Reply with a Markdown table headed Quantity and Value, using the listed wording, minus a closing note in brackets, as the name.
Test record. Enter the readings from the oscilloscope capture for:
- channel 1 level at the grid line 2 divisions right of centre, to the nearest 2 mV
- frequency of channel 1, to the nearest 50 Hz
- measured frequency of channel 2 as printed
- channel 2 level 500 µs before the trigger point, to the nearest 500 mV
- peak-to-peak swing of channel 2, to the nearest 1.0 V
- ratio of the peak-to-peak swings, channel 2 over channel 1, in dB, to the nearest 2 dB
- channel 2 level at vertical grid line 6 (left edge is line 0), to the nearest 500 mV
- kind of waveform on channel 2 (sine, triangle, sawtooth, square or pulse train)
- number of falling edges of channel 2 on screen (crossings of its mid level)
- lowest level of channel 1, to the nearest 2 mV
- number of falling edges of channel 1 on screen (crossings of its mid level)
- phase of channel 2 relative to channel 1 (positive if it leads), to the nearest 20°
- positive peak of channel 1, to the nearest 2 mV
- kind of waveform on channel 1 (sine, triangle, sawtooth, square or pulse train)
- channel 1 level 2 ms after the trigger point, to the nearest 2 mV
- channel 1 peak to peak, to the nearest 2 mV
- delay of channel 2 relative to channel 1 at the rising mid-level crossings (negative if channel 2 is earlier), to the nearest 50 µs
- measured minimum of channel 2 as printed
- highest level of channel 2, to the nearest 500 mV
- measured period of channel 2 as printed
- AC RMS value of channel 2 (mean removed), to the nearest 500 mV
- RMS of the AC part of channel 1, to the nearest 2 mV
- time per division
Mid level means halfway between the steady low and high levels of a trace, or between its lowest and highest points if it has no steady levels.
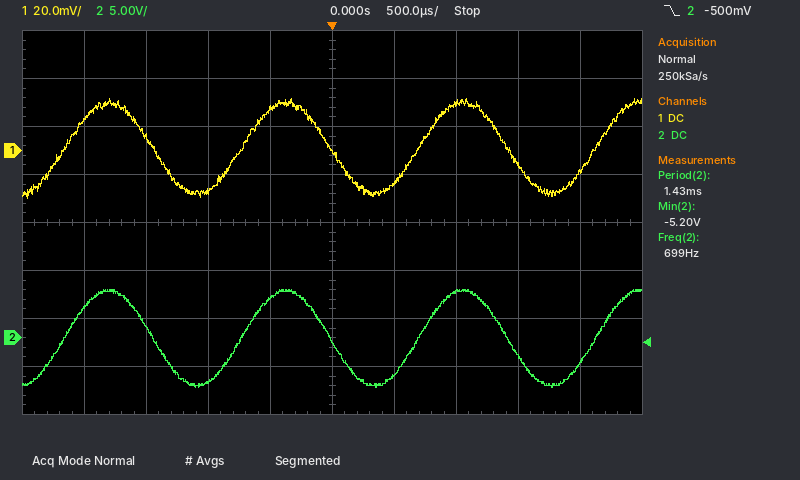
| Quantity | Value |
|---|---|
| channel 1 level at the grid line 2 divisions right of centre, to the nearest 2 mV | 20 mV |
| frequency of channel 1, to the nearest 50 Hz | 700 Hz |
| measured frequency of channel 2 as printed | 699 Hz |
| channel 2 level 500 µs before the trigger point, to the nearest 500 mV | 4.0 V |
| peak-to-peak swing of channel 2, to the nearest 1.0 V | 10.0 V |
| ratio of the peak-to-peak swings, channel 2 over channel 1, in dB, to the nearest 2 dB | 48 dB |
| channel 2 level at vertical grid line 6 (left edge is line 0), to the nearest 500 mV | -4.0 V |
| kind of waveform on channel 2 | sine |
| number of falling edges of channel 2 on screen | 3 |
| lowest level of channel 1, to the nearest 2 mV | -20 mV |
| number of falling edges of channel 1 on screen | 3 |
| phase of channel 2 relative to channel 1 (positive if it leads), to the nearest 20° | 0° |
| positive peak of channel 1, to the nearest 2 mV | 22 mV |
| kind of waveform on channel 1 | sine |
| channel 1 level 2 ms after the trigger point, to the nearest 2 mV | -8 mV |
| channel 1 peak to peak, to the nearest 2 mV | 42 mV |
| delay of channel 2 relative to channel 1 at the rising mid-level crossings (negative if channel 2 is earlier), to the nearest 50 µs | 0 µs |
| measured minimum of channel 2 as printed | -5.20 V |
| highest level of channel 2, to the nearest 500 mV | 5.0 V |
| measured period of channel 2 as printed | 1.43 ms |
| AC RMS value of channel 2 (mean removed), to the nearest 500 mV | 3.5 V |
| RMS of the AC part of channel 1, to the nearest 2 mV | 14 mV |
| time per division | 500 µs |
